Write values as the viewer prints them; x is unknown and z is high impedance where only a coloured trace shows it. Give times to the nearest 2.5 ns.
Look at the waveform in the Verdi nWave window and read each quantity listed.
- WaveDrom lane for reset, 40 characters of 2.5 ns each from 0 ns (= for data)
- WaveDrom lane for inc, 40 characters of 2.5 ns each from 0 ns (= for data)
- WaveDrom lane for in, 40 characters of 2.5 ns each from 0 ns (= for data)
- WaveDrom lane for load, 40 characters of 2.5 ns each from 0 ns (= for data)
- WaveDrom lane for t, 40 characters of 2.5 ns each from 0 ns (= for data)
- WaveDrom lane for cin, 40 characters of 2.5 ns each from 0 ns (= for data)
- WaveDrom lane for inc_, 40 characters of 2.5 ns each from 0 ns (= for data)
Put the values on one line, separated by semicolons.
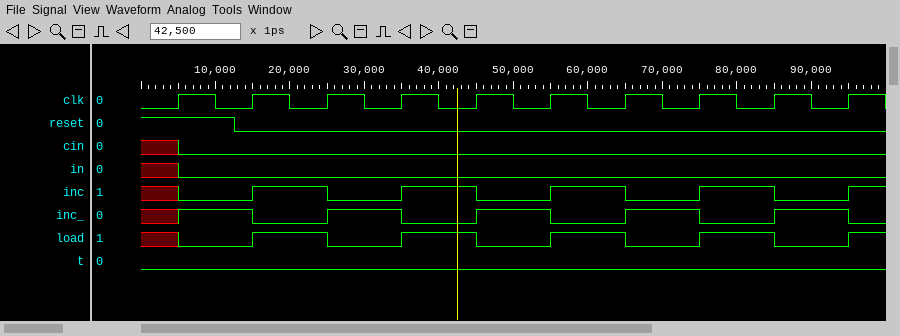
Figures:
{name: 'reset', wave: '1....0..................................'}; {name: 'inc', wave: 'x.0...1...0...1...0...1...0...1...0...1.'}; {name: 'in', wave: 'x.0.....................................'}; {name: 'load', wave: 'x.0...1...0...1...0...1...0...1...0...1.'}; {name: 't', wave: '0.......................................'}; {name: 'cin', wave: 'x.0.....................................'}; {name: 'inc_', wave: 'x.1...0...1...0...1...0...1...0...1...0.'}
